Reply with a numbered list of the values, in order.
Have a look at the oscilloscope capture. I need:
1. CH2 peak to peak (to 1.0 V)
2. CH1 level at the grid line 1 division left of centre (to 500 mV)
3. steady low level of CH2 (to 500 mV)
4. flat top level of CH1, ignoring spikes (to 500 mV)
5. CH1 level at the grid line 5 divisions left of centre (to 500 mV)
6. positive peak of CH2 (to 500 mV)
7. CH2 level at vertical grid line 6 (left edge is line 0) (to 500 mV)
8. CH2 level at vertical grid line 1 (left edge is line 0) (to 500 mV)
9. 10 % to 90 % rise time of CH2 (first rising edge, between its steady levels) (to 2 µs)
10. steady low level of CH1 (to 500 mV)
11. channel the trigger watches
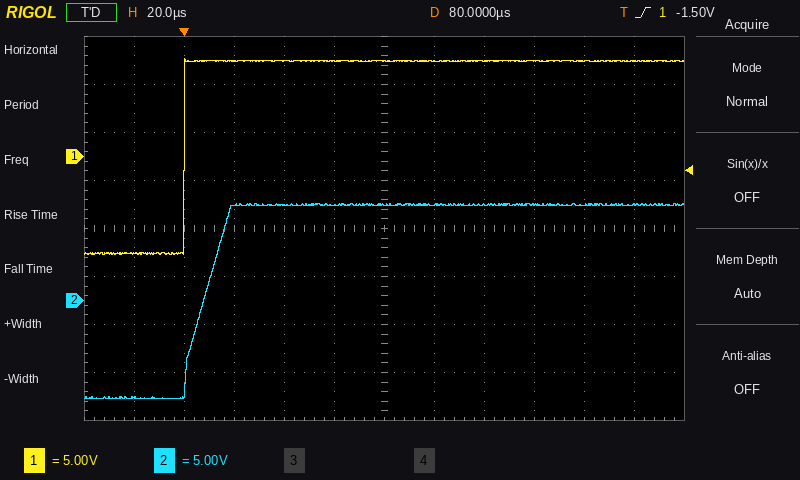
1. 20.0 V
2. 10.0 V
3. -10.0 V
4. 10.0 V
5. -10.0 V
6. 10.0 V
7. 10.0 V
8. -10.0 V
9. 16 µs
10. -10.0 V
11. CH1
